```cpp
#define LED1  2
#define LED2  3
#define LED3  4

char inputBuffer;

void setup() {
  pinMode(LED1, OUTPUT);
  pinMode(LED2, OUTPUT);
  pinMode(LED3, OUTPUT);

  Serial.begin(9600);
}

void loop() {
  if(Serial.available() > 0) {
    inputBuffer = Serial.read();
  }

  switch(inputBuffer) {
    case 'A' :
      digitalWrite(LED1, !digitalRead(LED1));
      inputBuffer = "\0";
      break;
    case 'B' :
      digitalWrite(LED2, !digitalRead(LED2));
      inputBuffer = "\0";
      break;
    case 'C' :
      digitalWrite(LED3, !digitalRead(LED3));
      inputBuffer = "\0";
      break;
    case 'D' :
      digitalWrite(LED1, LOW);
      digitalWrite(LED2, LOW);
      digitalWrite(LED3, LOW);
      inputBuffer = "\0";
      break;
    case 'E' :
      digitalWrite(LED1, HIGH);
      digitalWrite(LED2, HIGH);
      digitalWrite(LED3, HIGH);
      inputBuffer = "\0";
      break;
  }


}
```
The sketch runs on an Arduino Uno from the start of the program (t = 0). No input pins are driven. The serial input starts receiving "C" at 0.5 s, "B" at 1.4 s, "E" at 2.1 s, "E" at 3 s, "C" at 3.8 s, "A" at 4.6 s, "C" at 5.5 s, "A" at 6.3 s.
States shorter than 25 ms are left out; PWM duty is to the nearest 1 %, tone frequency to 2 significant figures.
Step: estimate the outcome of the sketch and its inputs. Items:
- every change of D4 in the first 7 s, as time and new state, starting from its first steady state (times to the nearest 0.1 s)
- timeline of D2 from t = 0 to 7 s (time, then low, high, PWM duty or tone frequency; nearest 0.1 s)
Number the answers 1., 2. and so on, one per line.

1. 0 s low; 0.5 s high; 3.8 s low; 5.5 s high
2. 0 s low; 2.1 s high; 4.6 s low; 6.3 s high
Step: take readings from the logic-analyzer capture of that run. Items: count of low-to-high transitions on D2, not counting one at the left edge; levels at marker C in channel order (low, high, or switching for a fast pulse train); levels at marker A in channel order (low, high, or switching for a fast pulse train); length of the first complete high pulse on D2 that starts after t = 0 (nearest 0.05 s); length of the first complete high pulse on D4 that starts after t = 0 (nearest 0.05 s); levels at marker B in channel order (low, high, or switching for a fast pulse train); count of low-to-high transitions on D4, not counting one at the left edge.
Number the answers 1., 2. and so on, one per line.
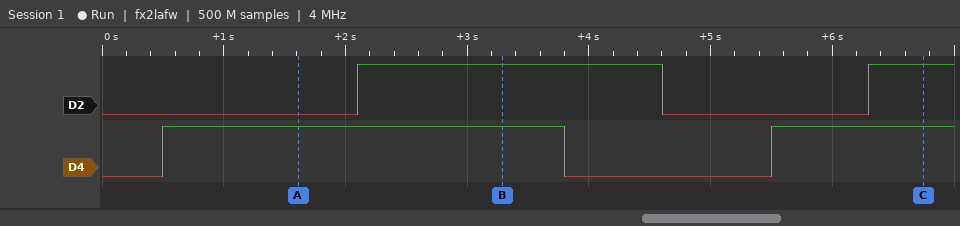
1. 2
2. D2 high, D4 high
3. D2 low, D4 high
4. 2.50 s
5. 3.30 s
6. D2 high, D4 high
7. 2
